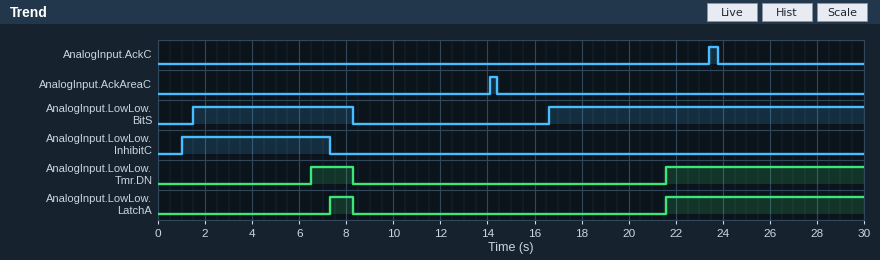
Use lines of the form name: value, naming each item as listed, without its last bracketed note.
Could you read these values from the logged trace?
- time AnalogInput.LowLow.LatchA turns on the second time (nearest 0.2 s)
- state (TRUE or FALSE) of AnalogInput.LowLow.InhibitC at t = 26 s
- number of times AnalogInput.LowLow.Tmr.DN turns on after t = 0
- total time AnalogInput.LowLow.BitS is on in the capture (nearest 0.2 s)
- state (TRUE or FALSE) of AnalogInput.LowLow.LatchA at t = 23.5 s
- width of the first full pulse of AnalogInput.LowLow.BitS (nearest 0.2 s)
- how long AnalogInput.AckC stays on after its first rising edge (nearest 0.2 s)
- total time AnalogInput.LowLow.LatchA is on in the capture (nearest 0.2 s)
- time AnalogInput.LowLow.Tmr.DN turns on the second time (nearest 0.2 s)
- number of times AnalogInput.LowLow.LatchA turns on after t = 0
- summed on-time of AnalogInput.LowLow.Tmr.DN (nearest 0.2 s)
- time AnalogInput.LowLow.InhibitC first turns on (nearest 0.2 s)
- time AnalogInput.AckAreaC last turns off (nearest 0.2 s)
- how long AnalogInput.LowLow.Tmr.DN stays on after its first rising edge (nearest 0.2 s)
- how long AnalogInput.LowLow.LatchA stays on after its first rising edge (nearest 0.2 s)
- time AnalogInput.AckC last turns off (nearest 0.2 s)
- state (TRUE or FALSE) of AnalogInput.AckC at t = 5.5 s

time AnalogInput.LowLow.LatchA turns on the second time: 21.6 s
state (TRUE or FALSE) of AnalogInput.LowLow.InhibitC at t = 26 s: FALSE
number of times AnalogInput.LowLow.Tmr.DN turns on after t = 0: 2
total time AnalogInput.LowLow.BitS is on in the capture: 20.2 s
state (TRUE or FALSE) of AnalogInput.LowLow.LatchA at t = 23.5 s: TRUE
width of the first full pulse of AnalogInput.LowLow.BitS: 6.8 s
how long AnalogInput.AckC stays on after its first rising edge: 0.4 s
total time AnalogInput.LowLow.LatchA is on in the capture: 9.4 s
time AnalogInput.LowLow.Tmr.DN turns on the second time: 21.6 s
number of times AnalogInput.LowLow.LatchA turns on after t = 0: 2
summed on-time of AnalogInput.LowLow.Tmr.DN: 10.2 s
time AnalogInput.LowLow.InhibitC first turns on: 1.0 s
time AnalogInput.AckAreaC last turns off: 14.4 s
how long AnalogInput.LowLow.Tmr.DN stays on after its first rising edge: 1.8 s
how long AnalogInput.LowLow.LatchA stays on after its first rising edge: 1.0 s
time AnalogInput.AckC last turns off: 23.8 s
state (TRUE or FALSE) of AnalogInput.AckC at t = 5.5 s: FALSE
